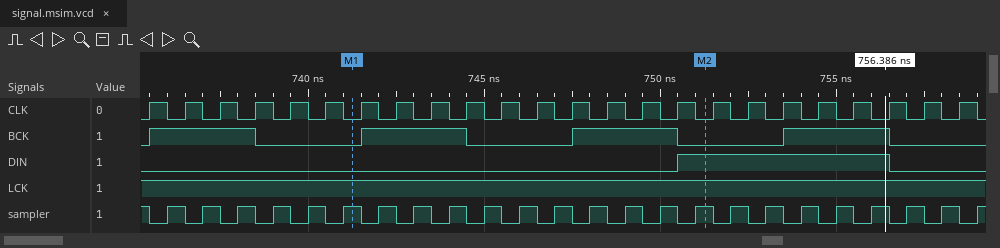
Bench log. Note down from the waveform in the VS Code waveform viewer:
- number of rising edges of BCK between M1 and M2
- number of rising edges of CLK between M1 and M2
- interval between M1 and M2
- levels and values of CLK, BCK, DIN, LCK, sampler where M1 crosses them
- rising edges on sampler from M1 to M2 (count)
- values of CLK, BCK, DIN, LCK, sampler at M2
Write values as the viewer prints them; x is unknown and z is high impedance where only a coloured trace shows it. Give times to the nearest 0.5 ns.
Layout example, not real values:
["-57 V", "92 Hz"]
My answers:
["2", "10", "10 ns", "CLK=0, BCK=0, DIN=0, LCK=1, sampler=1", "10", "CLK=0, BCK=0, DIN=1, LCK=1, sampler=1"]
